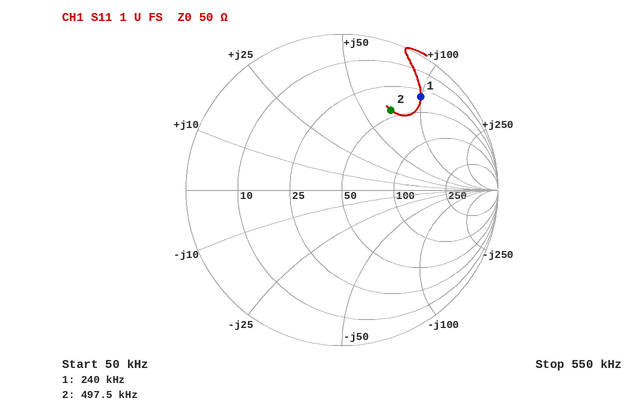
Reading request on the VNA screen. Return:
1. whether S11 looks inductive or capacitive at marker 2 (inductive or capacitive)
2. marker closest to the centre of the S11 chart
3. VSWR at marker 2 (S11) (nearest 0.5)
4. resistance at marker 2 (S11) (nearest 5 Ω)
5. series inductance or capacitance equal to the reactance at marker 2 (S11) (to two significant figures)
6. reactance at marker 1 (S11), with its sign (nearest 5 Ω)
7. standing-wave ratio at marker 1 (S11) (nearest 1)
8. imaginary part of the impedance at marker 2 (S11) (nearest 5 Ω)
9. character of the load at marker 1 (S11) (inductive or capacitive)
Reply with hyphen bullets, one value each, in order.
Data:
- inductive
- marker 2
- 4.0
- 45 Ω
- 22 µH
- +100 Ω
- 8
- +70 Ω
- inductive
